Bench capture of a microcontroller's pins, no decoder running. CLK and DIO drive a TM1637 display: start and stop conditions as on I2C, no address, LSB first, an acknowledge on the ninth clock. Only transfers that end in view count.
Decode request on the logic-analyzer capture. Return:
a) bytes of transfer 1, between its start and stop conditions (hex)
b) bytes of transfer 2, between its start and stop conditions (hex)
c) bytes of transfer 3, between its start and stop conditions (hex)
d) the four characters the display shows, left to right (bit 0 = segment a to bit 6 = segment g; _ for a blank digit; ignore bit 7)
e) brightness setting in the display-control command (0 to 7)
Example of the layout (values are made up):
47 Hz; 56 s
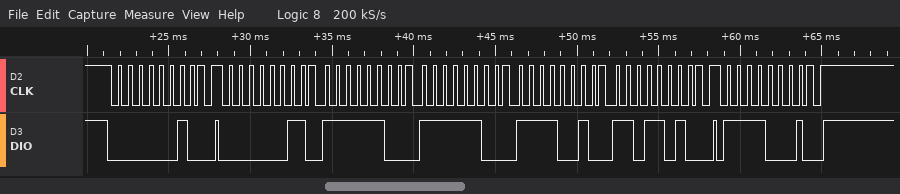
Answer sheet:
40; C0 3F 3F 4F 5B; 8F; 0032; 7
